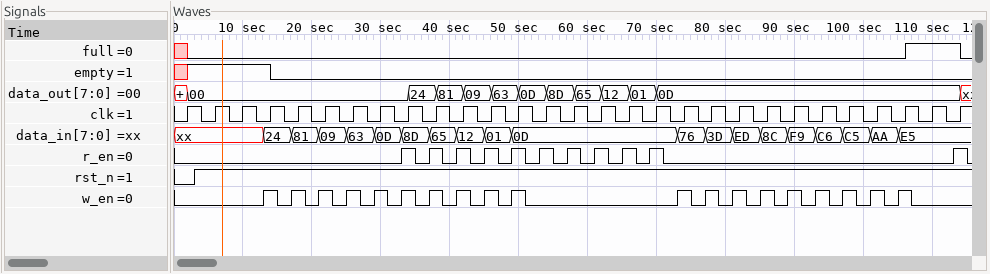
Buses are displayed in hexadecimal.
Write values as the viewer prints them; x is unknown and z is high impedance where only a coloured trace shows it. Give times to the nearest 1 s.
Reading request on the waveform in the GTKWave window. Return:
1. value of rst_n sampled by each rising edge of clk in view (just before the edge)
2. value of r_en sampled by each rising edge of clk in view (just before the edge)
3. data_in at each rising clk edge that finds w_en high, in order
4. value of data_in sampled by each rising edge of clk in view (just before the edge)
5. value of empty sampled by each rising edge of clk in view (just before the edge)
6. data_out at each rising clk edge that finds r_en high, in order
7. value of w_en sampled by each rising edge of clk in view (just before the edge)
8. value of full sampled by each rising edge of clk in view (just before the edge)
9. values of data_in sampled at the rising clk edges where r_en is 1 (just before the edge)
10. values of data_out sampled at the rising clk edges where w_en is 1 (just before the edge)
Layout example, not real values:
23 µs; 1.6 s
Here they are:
0 1 1 1 1 1 1 1 1 1 1 1 1 1 1 1 1 1 1 1 1 1 1 1 1 1 1 1 1; 0 0 0 0 0 0 0 0 1 1 1 1 1 1 1 1 1 1 0 0 0 0 0 0 0 0 0 0 1; 24, 81, 09, 63, 0D, 8D, 65, 12, 01, 0D, 76, 3D, ED, 8C, F9, C6, C5, AA, E5; xx, xx, xx, 24, 81, 09, 63, 0D, 8D, 65, 12, 01, 0D, 0D, 0D, 0D, 0D, 0D, 76, 3D, ED, 8C, F9, C6, C5, AA, E5, E5, E5; x 1 1 1 0 0 0 0 0 0 0 0 0 0 0 0 0 0 0 0 0 0 0 0 0 0 0 0 0; 00, 24, 81, 09, 63, 0D, 8D, 65, 12, 01, 0D; 0 0 0 1 1 1 1 1 1 1 1 1 1 0 0 0 0 0 1 1 1 1 1 1 1 1 1 0 0; x 0 0 0 0 0 0 0 0 0 0 0 0 0 0 0 0 0 0 0 0 0 0 0 0 0 0 1 1; 8D, 65, 12, 01, 0D, 0D, 0D, 0D, 0D, 0D, E5; 00, 00, 00, 00, 00, 00, 24, 81, 09, 63, 0D, 0D, 0D, 0D, 0D, 0D, 0D, 0D, 0D
